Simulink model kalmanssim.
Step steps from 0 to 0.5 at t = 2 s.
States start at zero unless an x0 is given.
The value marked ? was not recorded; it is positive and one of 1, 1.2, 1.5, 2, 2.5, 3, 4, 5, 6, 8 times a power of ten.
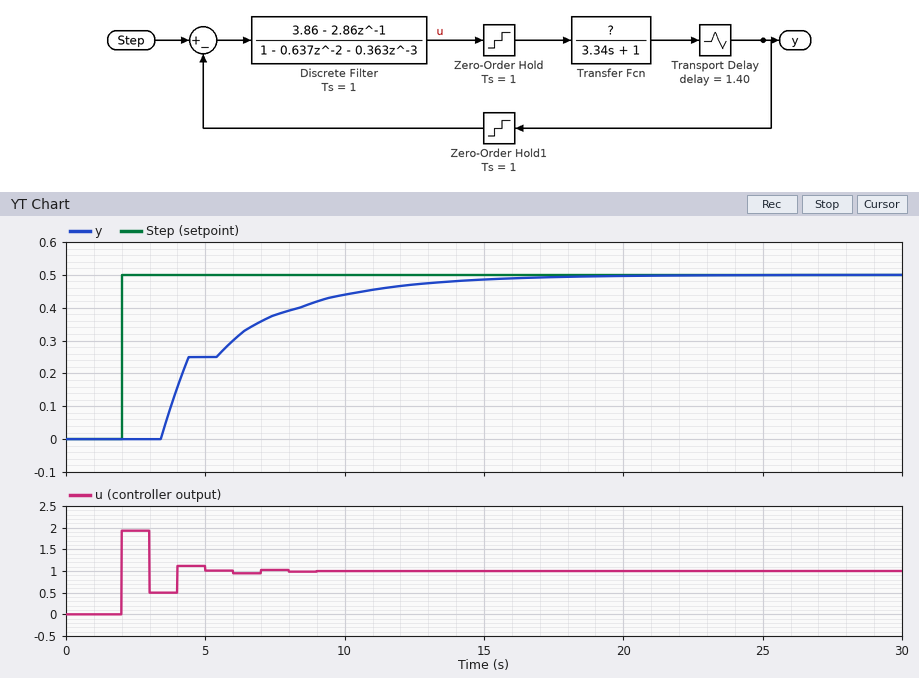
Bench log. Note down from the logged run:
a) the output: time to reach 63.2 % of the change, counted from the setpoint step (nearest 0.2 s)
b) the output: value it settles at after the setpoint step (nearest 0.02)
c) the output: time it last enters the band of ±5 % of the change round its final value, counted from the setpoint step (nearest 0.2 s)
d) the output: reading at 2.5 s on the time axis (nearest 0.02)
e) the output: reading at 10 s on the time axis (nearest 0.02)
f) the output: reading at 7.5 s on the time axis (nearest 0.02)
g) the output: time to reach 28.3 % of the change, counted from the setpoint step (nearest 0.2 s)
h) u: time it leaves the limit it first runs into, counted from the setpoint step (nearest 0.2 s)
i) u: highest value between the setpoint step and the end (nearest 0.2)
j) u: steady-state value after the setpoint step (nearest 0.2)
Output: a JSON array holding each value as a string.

["4.2 s", "0.50", "11.0 s", "0.00", "0.44", "0.38", "2.0 s", "1.0 s", "2.0", "1.0"]
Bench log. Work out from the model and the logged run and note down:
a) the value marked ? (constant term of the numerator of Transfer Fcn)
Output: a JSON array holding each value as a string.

["0.5"]
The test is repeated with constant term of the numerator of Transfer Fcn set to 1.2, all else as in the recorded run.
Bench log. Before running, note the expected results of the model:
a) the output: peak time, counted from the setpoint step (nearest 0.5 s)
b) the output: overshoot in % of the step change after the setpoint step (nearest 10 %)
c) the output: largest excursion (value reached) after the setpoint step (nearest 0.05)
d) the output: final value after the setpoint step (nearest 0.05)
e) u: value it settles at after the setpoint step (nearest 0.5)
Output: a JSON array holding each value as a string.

["3.5 s", "20 %", "0.60", "0.50", "0.5"]
